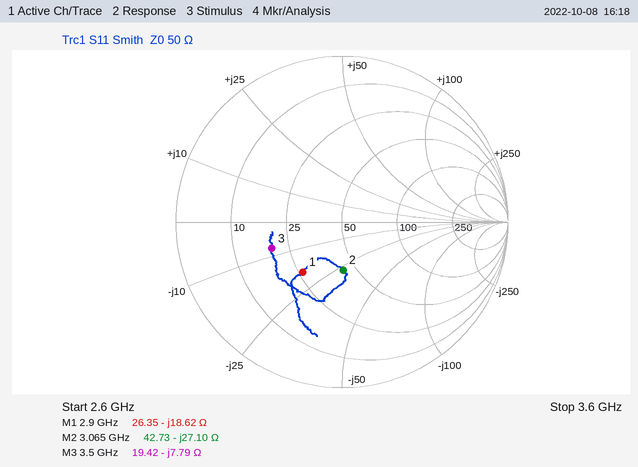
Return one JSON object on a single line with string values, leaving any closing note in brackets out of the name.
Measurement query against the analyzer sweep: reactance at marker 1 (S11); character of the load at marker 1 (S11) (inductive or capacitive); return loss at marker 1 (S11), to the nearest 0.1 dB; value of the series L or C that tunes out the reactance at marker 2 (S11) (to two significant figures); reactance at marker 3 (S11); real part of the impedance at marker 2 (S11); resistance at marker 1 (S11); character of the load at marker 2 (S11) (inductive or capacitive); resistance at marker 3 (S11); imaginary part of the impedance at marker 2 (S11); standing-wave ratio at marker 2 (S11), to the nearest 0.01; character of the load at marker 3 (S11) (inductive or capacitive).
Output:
{"reactance at marker 1": "-18.62 Ω", "character of the load at marker 1 (S11)": "capacitive", "return loss at marker 1 (S11), to the nearest 0.1 dB": "8.3 dB", "value of the series L or C that tunes out the reactance at marker 2 (S11)": "1.4 nH", "reactance at marker 3": "-7.79 Ω", "real part of the impedance at marker 2": "42.73 Ω", "resistance at marker 1": "26.35 Ω", "character of the load at marker 2 (S11)": "capacitive", "resistance at marker 3": "19.42 Ω", "imaginary part of the impedance at marker 2": "-27.10 Ω", "standing-wave ratio at marker 2 (S11), to the nearest 0.01": "1.82", "character of the load at marker 3 (S11)": "capacitive"}
